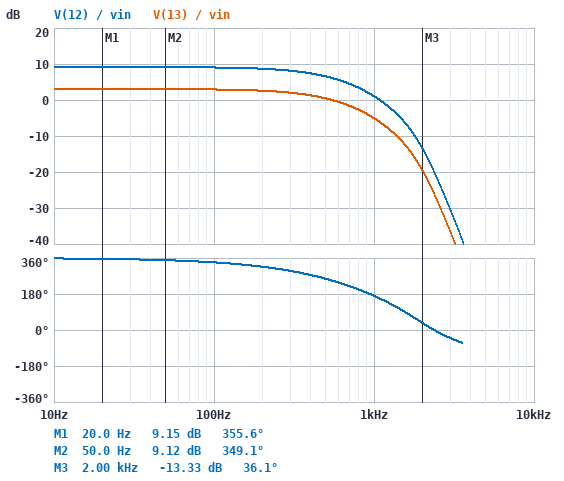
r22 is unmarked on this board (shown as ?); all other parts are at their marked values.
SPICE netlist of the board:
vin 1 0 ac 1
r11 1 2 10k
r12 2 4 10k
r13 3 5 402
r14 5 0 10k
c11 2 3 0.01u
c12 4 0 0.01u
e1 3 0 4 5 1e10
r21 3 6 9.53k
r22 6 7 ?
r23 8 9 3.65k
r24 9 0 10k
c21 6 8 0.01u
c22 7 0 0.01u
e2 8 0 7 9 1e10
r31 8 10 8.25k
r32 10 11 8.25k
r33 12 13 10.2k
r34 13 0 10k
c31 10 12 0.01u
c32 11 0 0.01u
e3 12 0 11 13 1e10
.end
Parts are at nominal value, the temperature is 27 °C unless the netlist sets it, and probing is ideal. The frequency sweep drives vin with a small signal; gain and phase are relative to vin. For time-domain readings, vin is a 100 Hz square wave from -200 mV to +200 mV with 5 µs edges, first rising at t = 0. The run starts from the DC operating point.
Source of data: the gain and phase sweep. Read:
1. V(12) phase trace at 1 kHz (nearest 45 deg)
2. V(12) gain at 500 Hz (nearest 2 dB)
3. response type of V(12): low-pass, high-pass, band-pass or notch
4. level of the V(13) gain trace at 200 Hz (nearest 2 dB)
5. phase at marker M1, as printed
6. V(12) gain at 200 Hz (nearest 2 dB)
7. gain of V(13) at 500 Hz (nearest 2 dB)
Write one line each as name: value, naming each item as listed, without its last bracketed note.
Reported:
V(12) phase trace at 1 kHz: 180 deg
V(12) gain at 500 Hz: 6 dB
response type of V(12): low-pass, high-pass, band-pass or notch: low-pass
level of the V(13) gain trace at 200 Hz: 2 dB
phase at marker M1, as printed: 355.6 deg
V(12) gain at 200 Hz: 8 dB
gain of V(13) at 500 Hz: 0 dB
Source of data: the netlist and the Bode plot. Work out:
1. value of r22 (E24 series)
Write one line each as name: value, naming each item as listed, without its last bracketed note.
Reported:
value of r22: 27 kΩ
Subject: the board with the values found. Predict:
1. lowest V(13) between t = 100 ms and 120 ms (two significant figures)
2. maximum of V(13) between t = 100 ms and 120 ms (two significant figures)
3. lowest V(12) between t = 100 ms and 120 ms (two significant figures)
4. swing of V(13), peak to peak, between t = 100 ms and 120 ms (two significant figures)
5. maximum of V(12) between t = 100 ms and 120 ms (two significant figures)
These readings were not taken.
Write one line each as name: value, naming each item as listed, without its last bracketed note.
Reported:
lowest V(13) between t = 100 ms and 120 ms: -280 mV
maximum of V(13) between t = 100 ms and 120 ms: 280 mV
lowest V(12) between t = 100 ms and 120 ms: -570 mV
swing of V(13), peak to peak, between t = 100 ms and 120 ms: 570 mV
maximum of V(12) between t = 100 ms and 120 ms: 570 mV
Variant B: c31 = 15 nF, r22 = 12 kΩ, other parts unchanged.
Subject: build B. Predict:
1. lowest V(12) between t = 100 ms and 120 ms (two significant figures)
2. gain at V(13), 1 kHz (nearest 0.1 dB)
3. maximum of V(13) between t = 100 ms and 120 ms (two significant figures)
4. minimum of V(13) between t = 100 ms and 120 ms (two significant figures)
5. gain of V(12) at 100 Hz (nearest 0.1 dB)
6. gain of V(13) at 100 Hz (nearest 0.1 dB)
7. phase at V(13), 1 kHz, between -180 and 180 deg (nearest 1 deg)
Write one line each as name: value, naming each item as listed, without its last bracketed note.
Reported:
lowest V(12) between t = 100 ms and 120 ms: -690 mV
gain at V(13), 1 kHz: 2.1 dB
maximum of V(13) between t = 100 ms and 120 ms: 340 mV
minimum of V(13) between t = 100 ms and 120 ms: -340 mV
gain of V(12) at 100 Hz: 9.1 dB
gain of V(13) at 100 Hz: 3.0 dB
phase at V(13), 1 kHz, between -180 and 180 deg: -150 deg
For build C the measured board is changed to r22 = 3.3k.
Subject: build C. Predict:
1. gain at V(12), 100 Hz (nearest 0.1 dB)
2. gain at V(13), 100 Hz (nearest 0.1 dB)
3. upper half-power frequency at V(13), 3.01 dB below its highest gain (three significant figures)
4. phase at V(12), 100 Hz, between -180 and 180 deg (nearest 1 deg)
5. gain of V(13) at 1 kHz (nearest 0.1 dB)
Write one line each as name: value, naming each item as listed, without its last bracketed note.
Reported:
gain at V(12), 100 Hz: 9.1 dB
gain at V(13), 100 Hz: 3.0 dB
upper half-power frequency at V(13), 3.01 dB below its highest gain: 1.17 kHz
phase at V(12), 100 Hz, between -180 and 180 deg: -13 deg
gain of V(13) at 1 kHz: 0.8 dB
